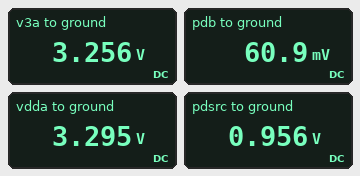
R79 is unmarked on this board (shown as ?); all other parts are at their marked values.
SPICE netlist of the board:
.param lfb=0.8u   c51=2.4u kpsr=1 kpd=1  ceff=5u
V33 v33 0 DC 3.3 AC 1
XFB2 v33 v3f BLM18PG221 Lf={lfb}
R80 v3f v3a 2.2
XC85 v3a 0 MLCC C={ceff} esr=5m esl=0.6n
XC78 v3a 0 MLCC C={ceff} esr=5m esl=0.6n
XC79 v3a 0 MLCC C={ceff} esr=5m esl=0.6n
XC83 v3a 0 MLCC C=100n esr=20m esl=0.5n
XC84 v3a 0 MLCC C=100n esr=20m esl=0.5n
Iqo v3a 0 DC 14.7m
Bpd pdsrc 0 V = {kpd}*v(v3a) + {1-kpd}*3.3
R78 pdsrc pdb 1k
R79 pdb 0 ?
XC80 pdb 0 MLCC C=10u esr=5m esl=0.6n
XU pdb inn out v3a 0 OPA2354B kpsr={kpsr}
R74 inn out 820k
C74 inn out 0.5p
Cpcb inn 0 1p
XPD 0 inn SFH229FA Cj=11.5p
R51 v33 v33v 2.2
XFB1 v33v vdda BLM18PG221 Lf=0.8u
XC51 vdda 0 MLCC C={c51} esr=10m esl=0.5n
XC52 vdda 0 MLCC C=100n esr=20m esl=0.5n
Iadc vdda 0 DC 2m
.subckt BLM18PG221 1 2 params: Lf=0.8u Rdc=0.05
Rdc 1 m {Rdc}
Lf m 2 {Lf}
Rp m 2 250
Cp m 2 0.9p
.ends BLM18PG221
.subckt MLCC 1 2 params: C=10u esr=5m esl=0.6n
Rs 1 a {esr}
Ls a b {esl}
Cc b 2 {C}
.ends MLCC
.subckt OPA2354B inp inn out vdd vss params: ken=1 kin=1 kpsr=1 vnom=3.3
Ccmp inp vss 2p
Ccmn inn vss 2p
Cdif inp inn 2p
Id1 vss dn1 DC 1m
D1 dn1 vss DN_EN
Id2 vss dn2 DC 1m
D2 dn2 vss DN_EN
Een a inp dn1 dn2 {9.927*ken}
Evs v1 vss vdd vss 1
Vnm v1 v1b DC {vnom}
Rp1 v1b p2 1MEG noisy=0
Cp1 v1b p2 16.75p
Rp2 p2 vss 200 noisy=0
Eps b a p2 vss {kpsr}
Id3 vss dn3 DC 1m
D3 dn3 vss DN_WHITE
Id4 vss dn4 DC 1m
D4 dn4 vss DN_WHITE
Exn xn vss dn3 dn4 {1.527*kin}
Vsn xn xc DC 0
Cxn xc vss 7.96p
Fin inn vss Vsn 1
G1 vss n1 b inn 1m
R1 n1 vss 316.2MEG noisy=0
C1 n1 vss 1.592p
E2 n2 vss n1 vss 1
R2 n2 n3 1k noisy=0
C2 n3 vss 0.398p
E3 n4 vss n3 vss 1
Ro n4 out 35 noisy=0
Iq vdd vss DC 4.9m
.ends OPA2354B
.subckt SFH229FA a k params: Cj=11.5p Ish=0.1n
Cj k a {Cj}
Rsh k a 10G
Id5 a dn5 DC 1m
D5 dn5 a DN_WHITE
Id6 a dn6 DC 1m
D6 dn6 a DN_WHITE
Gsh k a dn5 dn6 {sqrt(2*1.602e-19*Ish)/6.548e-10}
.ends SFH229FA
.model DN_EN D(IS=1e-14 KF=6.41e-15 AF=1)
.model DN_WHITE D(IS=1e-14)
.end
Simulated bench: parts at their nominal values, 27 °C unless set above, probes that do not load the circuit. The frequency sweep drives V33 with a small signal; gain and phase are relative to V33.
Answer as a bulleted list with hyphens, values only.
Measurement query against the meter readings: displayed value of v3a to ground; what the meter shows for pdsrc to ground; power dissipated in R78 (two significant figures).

- 3.256 V
- 0.956 V
- 800 µW
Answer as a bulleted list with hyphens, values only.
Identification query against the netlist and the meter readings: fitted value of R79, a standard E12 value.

- 68 Ω
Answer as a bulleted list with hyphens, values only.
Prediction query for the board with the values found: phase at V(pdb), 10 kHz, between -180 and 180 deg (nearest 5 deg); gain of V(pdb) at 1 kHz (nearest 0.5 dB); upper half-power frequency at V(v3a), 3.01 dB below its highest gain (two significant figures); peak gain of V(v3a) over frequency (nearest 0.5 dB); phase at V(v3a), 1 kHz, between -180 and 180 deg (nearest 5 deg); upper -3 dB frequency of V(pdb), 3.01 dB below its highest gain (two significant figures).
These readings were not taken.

- -155 deg
- -36.5 dB
- 4.7 kHz
- 0 dB
- -10 deg
- 250 Hz
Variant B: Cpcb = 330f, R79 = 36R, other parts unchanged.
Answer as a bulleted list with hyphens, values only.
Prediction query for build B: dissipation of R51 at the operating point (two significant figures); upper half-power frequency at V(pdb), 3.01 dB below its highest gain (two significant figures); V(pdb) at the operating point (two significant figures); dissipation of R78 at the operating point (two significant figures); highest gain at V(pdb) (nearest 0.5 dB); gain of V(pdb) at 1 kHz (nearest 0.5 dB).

- 8.8 µW
- 450 Hz
- 33 mV
- 850 µW
- -29.0 dB
- -37.0 dB
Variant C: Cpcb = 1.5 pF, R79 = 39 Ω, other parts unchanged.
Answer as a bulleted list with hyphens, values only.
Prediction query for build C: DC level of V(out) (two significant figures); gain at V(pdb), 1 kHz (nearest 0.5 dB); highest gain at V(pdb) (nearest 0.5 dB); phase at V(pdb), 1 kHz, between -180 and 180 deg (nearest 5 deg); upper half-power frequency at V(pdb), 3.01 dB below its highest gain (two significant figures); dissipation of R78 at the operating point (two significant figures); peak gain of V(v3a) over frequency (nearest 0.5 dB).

- 36 mV
- -37.0 dB
- -28.5 dB
- -80 deg
- 420 Hz
- 850 µW
- 0 dB
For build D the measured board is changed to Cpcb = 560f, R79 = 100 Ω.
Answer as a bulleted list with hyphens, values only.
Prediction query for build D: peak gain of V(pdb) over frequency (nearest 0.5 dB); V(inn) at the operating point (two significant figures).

- -21.0 dB
- 87 mV
